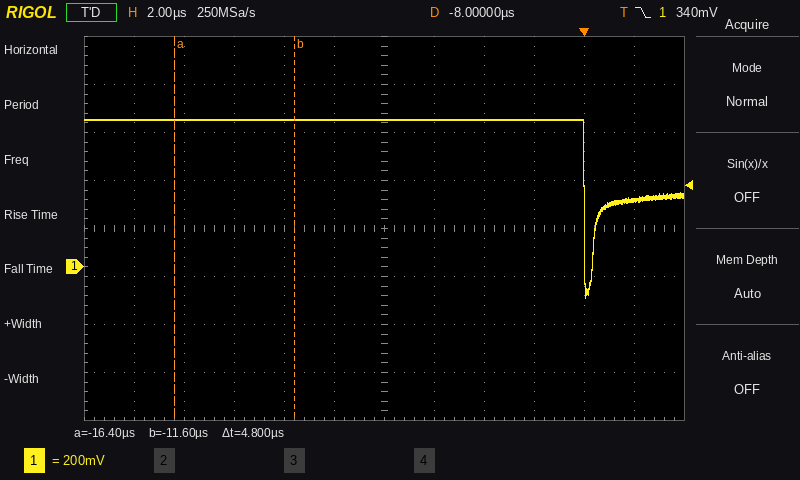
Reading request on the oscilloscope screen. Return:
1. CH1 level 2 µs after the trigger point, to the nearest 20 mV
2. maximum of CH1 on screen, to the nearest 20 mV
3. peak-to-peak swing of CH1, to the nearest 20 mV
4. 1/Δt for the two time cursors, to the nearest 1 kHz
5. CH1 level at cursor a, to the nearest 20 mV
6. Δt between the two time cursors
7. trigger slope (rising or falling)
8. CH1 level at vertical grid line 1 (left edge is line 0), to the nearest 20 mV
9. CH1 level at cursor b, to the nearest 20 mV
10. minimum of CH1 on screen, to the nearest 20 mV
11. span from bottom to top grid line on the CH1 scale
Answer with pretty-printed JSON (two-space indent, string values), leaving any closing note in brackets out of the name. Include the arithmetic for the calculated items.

{
  "CH1 level 2 µs after the trigger point, to the nearest 20 mV": "280 mV",
  "maximum of CH1 on screen, to the nearest 20 mV": "620 mV",
  "peak-to-peak swing of CH1, to the nearest 20 mV": "620 mV − (-120 mV) = 740 mV",
  "1/Δt for the two time cursors, to the nearest 1 kHz": "1 / 4.8 µs ≈ 208 kHz",
  "CH1 level at cursor a, to the nearest 20 mV": "620 mV",
  "Δt between the two time cursors": "4.8 µs",
  "trigger slope": "falling",
  "CH1 level at vertical grid line 1 (left edge is line 0), to the nearest 20 mV": "620 mV",
  "CH1 level at cursor b, to the nearest 20 mV": "620 mV",
  "minimum of CH1 on screen, to the nearest 20 mV": "-120 mV",
  "span from bottom to top grid line on the CH1 scale": "1.6 V"
}
